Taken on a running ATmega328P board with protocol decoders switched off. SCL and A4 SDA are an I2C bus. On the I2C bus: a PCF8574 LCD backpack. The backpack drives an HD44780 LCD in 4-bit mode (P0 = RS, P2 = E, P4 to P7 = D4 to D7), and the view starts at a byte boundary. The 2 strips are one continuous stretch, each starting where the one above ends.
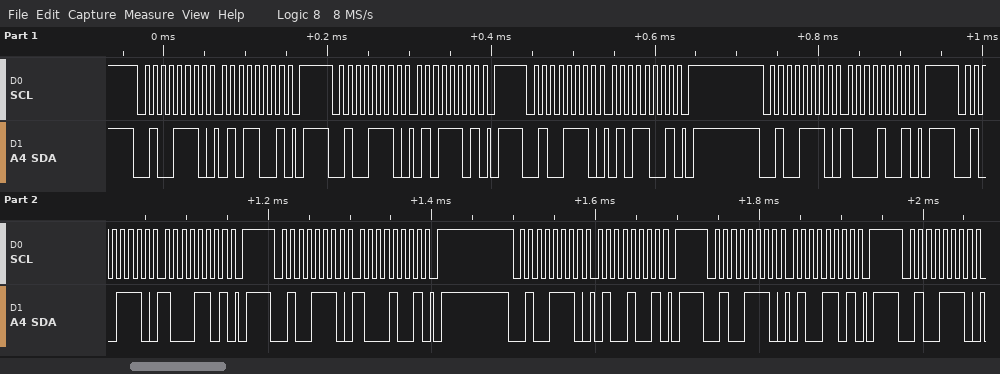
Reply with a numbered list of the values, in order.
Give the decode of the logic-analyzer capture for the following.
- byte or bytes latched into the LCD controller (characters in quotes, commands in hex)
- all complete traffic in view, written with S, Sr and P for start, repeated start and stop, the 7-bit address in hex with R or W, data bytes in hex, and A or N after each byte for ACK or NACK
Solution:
1. 'X'
2. S 27W A 59 A P S 27W A 5D A P S 27W A 59 A P S 27W A 89 A P S 27W A 8D A P S 27W A 89 A P S 27W A 49 A P S 27W A 4D A P S 27W A
